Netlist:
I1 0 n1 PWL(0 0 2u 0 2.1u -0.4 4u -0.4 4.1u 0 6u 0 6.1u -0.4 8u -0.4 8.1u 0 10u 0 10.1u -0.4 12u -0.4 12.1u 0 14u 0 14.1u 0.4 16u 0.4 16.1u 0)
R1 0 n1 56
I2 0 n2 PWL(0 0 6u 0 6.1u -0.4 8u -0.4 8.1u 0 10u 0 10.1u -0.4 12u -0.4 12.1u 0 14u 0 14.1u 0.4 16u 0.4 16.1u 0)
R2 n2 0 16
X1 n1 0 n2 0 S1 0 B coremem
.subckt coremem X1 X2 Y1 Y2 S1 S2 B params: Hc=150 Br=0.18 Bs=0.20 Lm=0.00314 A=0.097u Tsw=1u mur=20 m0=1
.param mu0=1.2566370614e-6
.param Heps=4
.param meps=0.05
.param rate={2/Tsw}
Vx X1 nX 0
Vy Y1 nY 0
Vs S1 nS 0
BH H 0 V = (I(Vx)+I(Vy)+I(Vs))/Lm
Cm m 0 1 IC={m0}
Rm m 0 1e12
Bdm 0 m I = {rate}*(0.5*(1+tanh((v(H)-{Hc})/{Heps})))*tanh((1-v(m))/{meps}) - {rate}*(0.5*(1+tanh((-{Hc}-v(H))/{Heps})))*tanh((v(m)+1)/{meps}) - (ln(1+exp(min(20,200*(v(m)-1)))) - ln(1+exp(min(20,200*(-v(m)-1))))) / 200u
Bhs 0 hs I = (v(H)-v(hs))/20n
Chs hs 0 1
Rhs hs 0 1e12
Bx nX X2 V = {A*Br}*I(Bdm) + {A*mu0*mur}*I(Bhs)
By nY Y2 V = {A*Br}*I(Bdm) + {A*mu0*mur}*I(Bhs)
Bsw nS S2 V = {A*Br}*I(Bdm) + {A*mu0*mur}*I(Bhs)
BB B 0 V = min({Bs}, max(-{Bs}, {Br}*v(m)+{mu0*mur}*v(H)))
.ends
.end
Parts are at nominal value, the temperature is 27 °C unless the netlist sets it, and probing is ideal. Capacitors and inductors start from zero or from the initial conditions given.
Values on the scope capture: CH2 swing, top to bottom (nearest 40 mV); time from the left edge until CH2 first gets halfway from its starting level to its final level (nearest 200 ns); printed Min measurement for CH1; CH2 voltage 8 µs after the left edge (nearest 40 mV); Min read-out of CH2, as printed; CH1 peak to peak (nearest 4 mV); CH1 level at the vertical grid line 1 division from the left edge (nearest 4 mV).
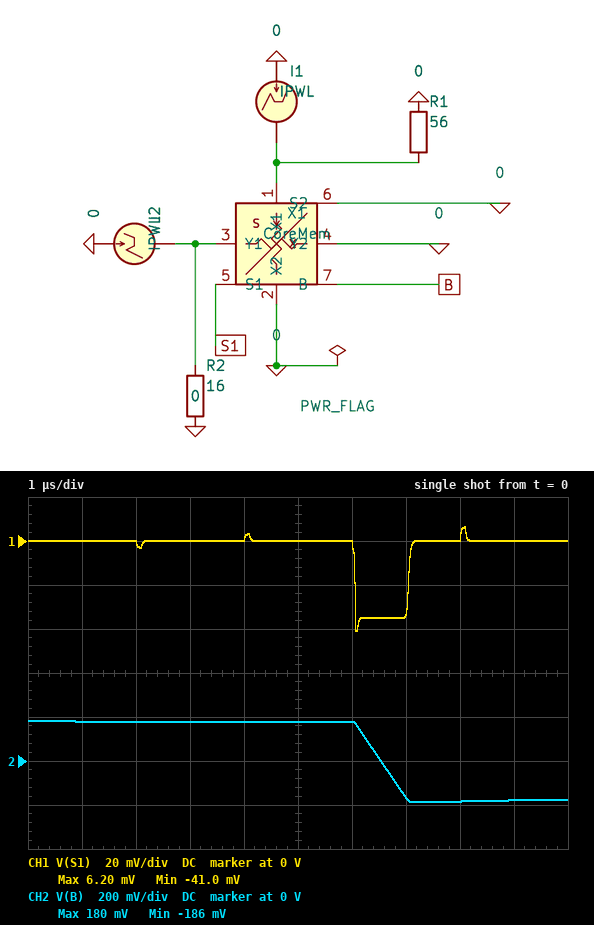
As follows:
360 mV
6.6 µs
-41.0 mV
-200 mV
-186 mV
48 mV
0 V
